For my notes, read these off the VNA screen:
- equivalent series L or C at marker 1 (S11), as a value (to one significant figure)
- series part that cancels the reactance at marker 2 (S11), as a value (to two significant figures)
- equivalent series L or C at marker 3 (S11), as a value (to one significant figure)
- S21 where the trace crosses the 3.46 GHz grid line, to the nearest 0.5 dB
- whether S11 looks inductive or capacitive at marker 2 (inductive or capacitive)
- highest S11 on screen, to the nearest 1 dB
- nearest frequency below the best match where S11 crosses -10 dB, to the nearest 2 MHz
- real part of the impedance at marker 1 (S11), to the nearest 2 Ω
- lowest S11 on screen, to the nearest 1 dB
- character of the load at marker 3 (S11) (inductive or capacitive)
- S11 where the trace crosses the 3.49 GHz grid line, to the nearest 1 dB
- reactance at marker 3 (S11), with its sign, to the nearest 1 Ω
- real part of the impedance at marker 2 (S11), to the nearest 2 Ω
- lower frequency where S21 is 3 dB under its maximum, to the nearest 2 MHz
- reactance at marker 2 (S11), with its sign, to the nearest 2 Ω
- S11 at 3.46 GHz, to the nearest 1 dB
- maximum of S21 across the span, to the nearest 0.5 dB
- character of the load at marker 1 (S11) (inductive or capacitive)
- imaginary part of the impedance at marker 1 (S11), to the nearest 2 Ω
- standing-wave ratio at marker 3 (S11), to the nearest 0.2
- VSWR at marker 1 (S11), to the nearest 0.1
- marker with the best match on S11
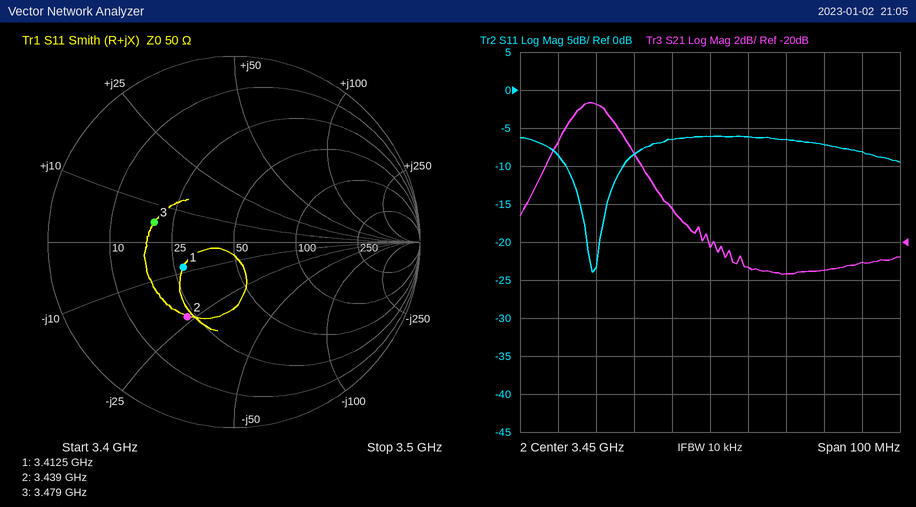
6 pF
1.1 nH
200 pH
-21.5 dB
capacitive
-6 dB
3.412 GHz
28 Ω
-24 dB
inductive
-8 dB
+5 Ω
22 Ω
3.408 GHz
-24 Ω
-6 dB
-12.5 dB
capacitive
-8 Ω
2.6
1.9
marker 1
